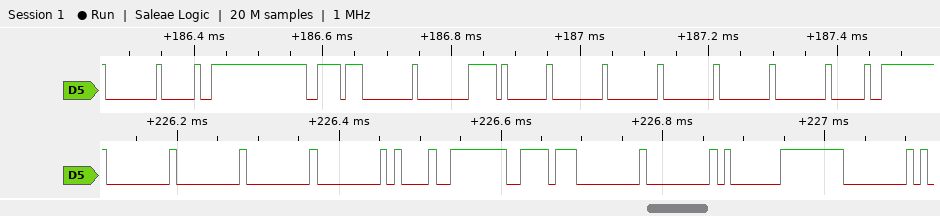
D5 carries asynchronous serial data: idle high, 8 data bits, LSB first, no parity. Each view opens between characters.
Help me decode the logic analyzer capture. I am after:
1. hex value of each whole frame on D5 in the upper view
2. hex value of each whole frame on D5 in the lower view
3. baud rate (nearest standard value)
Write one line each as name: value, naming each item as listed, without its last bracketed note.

hex value of each whole frame on D5 in the upper view: 00, 20, DE, 00, 00, 01, 00, 00, 00, 00, 00, 20
hex value of each whole frame on D5 in the lower view: 00, 00, 00, 00, 21, DE, 00, 00, 01, 00
baud rate: 115200 baud
